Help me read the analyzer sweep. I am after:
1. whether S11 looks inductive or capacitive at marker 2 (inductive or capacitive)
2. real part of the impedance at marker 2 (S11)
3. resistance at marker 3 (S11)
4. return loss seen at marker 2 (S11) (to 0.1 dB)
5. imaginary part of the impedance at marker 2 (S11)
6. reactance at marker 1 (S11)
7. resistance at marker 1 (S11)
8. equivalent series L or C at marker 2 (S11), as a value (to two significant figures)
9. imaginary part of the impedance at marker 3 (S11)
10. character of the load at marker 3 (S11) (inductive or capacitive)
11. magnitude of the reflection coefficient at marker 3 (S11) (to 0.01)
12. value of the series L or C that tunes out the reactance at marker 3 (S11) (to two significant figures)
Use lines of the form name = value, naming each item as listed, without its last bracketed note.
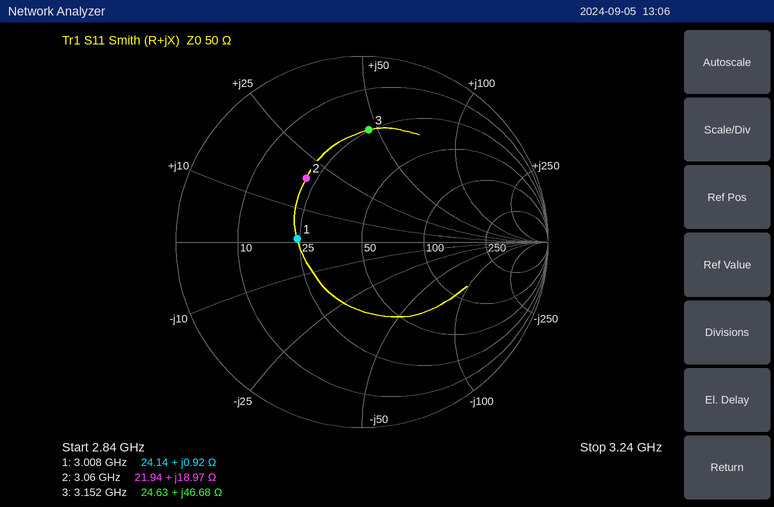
whether S11 looks inductive or capacitive at marker 2 = inductive
real part of the impedance at marker 2 = 21.94 Ω
resistance at marker 3 = 24.63 Ω
return loss seen at marker 2 (S11) = 6.8 dB
imaginary part of the impedance at marker 2 = +18.97 Ω
reactance at marker 1 = +0.92 Ω
resistance at marker 1 = 24.14 Ω
equivalent series L or C at marker 2 (S11), as a value = 990 pH
imaginary part of the impedance at marker 3 = +46.68 Ω
character of the load at marker 3 (S11) = inductive
magnitude of the reflection coefficient at marker 3 (S11) = 0.60
value of the series L or C that tunes out the reactance at marker 3 (S11) = 1.1 pF
